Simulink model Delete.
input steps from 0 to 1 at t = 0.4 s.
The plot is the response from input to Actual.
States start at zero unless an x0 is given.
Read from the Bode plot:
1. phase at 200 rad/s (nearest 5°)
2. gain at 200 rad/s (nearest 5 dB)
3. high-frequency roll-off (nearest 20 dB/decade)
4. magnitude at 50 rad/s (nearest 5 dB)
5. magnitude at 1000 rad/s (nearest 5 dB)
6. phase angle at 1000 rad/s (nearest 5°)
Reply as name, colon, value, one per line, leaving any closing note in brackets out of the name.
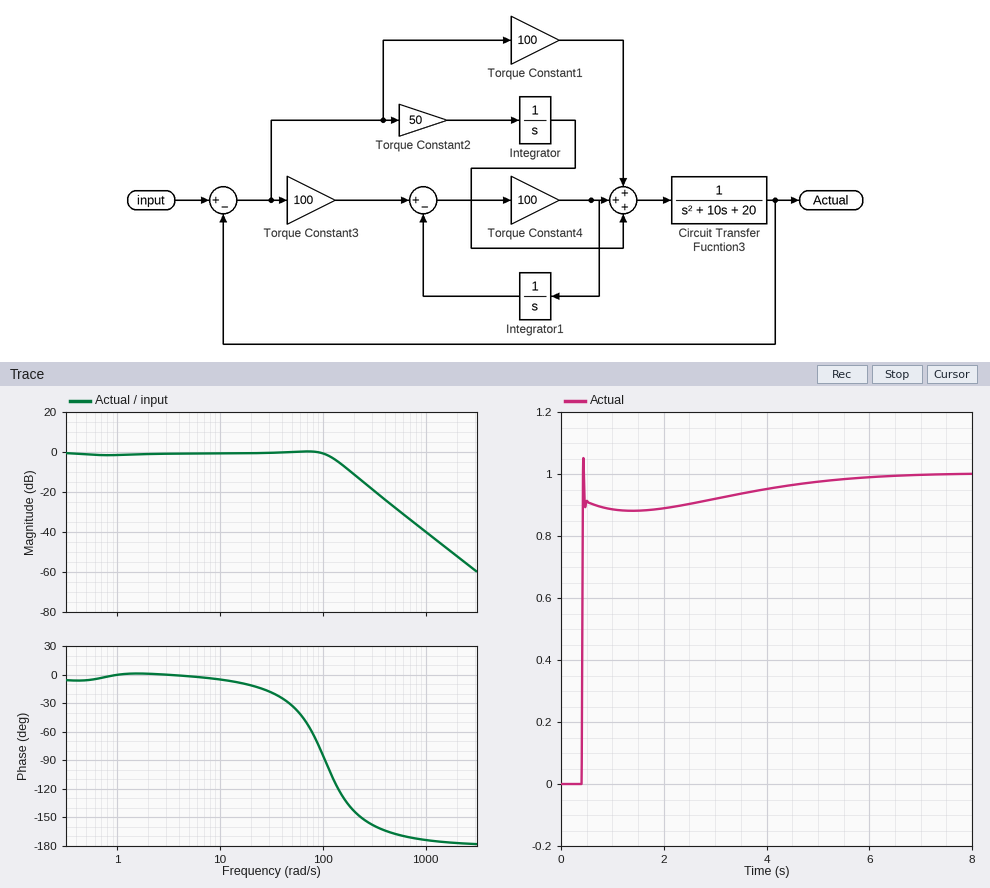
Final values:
phase at 200 rad/s: -145°
gain at 200 rad/s: -10 dB
high-frequency roll-off: -40 dB/decade
magnitude at 50 rad/s: 0 dB
magnitude at 1000 rad/s: -40 dB
phase angle at 1000 rad/s: -175°
